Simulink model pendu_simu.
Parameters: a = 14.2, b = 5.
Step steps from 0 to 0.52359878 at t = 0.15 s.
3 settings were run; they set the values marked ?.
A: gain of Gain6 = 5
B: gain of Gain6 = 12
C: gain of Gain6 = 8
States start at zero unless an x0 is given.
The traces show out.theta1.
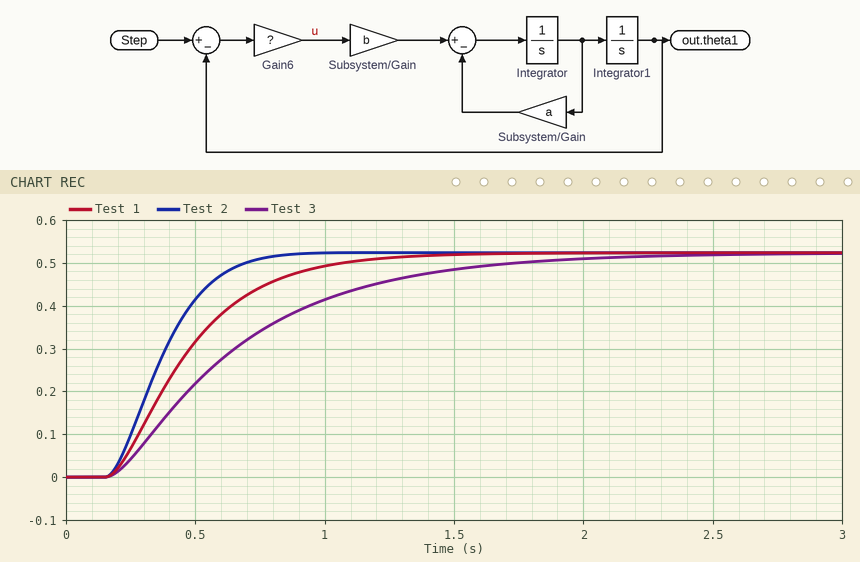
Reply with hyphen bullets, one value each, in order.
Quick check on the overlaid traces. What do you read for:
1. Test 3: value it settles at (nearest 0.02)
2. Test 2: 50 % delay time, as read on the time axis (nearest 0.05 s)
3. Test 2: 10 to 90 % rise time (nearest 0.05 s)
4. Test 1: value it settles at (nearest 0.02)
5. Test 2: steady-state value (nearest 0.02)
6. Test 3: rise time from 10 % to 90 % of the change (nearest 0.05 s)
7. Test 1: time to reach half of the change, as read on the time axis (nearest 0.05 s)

- 0.52
- 0.35 s
- 0.40 s
- 0.52
- 0.52
- 1.10 s
- 0.45 s
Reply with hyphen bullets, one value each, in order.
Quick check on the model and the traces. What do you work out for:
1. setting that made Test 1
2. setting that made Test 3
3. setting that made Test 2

- C
- A
- B
